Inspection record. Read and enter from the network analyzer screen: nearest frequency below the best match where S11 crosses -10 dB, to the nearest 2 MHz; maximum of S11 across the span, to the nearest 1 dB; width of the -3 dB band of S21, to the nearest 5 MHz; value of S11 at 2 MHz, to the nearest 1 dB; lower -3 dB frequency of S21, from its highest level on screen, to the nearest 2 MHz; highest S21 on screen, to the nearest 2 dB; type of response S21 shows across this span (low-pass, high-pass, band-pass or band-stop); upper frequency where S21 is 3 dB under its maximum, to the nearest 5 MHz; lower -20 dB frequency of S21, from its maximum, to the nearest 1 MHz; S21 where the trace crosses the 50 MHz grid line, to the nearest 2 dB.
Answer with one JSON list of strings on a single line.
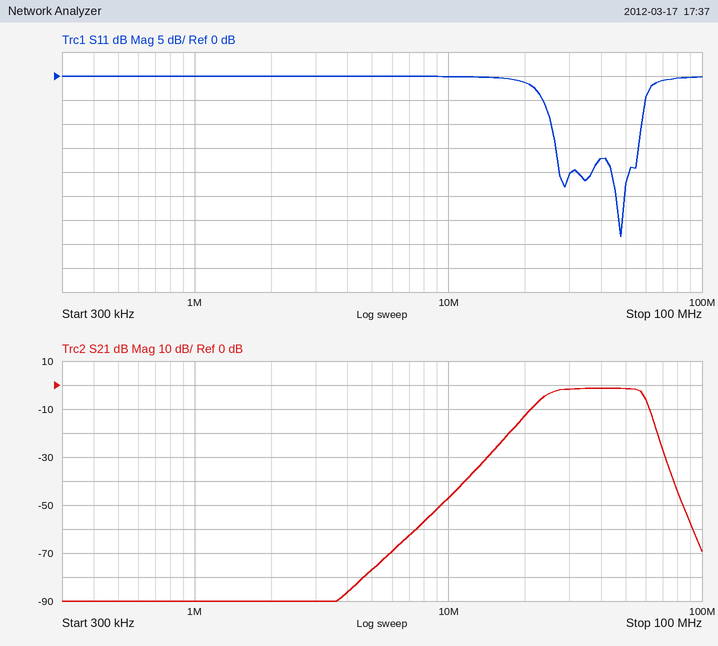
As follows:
["26 MHz", "0 dB", "35 MHz", "0 dB", "24 MHz", "-2 dB", "band-pass", "60 MHz", "17 MHz", "-2 dB"]
